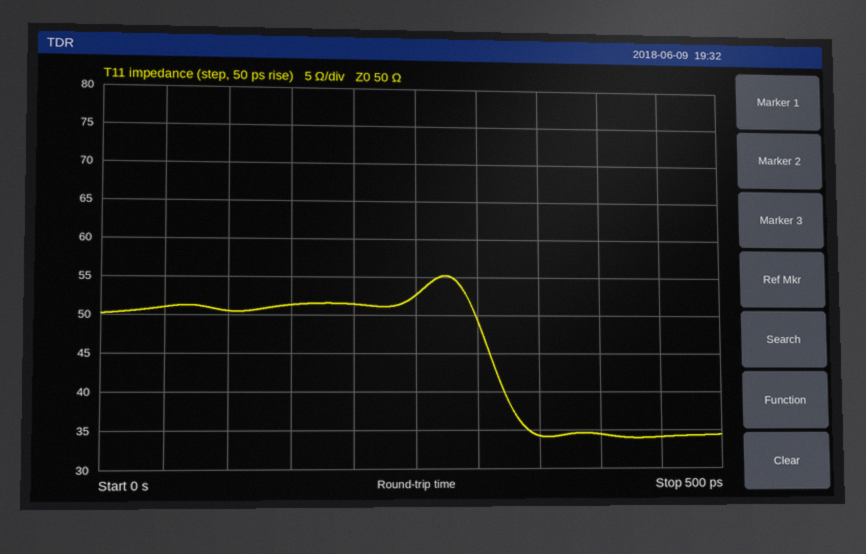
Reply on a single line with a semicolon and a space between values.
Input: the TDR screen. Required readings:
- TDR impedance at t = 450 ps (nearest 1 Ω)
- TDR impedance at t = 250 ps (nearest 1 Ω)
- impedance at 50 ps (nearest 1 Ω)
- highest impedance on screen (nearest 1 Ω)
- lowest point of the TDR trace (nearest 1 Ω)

34 Ω; 53 Ω; 51 Ω; 55 Ω; 34 Ω
